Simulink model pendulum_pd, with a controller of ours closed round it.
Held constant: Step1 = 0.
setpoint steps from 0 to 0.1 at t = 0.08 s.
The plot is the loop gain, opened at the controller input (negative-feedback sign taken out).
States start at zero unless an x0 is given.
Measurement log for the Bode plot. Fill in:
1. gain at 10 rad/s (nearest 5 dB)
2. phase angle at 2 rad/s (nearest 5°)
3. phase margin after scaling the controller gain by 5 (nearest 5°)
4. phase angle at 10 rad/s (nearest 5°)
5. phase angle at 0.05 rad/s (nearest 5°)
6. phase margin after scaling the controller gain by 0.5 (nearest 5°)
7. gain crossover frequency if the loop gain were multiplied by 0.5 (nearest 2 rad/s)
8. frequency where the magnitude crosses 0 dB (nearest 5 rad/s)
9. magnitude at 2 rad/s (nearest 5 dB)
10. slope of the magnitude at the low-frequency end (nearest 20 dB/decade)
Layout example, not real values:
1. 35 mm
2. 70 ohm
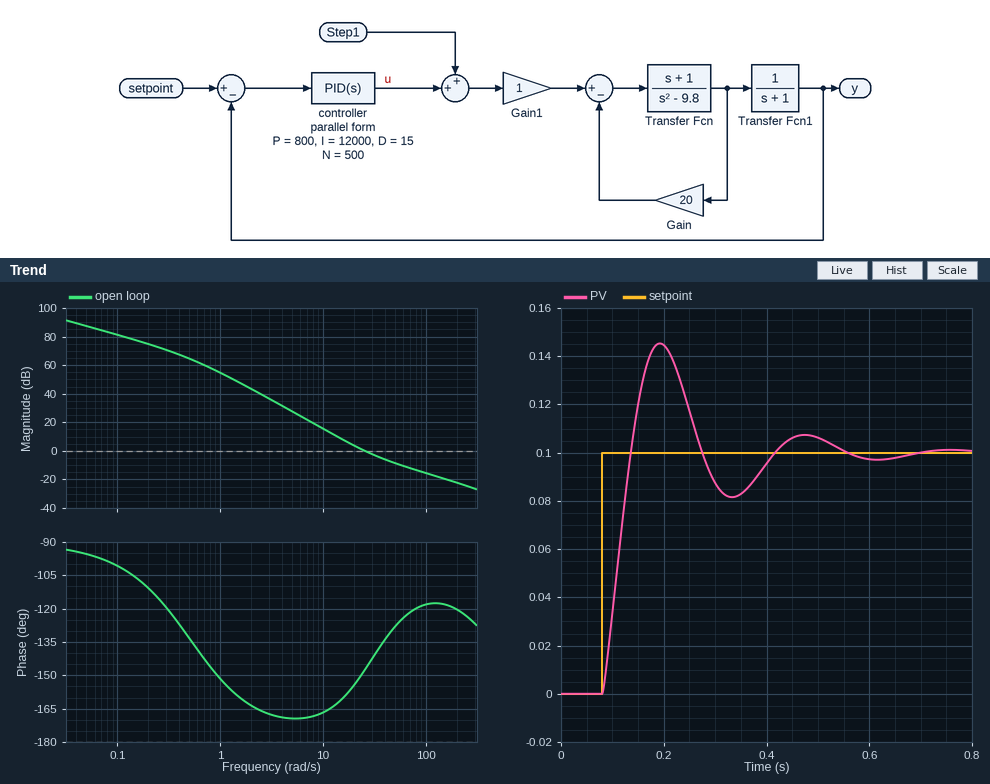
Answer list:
1. 15 dB
2. -165°
3. 60°
4. -165°
5. -95°
6. 20°
7. 18 rad/s
8. 25 rad/s
9. 45 dB
10. -20 dB/decade
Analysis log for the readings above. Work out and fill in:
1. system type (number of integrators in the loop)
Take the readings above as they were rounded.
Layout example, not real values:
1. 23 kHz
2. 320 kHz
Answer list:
1. 1
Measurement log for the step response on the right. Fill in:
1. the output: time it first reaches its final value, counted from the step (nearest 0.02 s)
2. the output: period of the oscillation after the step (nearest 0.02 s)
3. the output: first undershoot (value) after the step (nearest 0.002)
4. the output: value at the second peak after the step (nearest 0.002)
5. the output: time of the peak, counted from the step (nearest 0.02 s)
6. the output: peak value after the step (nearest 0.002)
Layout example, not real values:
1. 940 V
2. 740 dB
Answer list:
1. 0.06 s
2. 0.28 s
3. 0.082
4. 0.108
5. 0.12 s
6. 0.146
